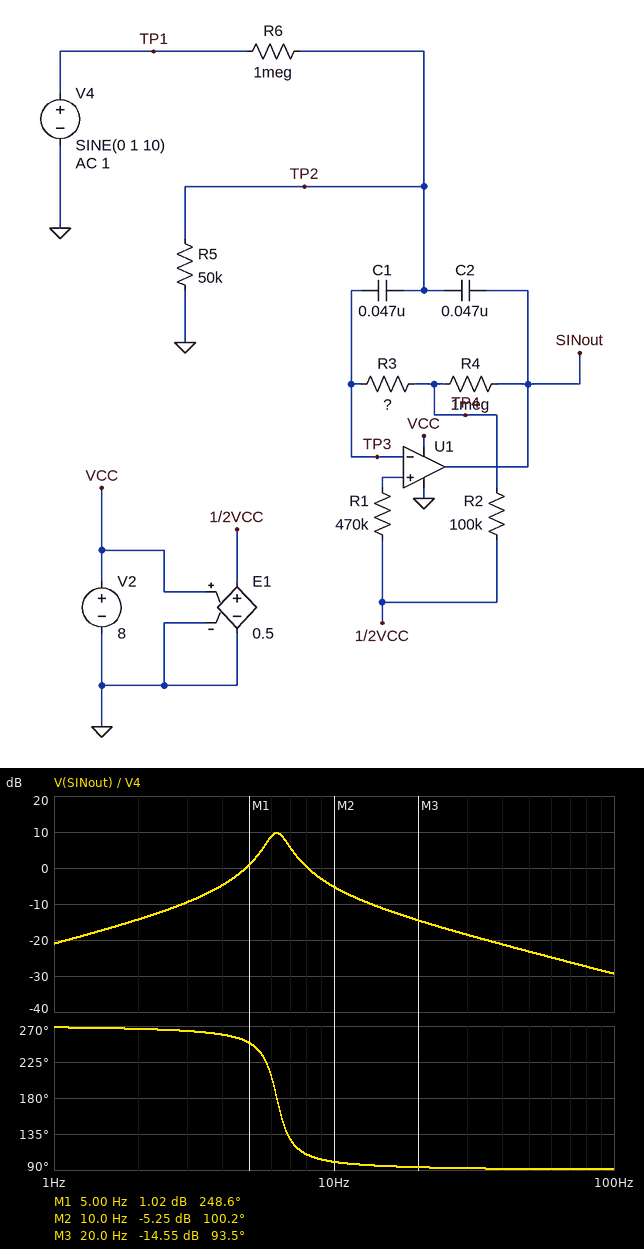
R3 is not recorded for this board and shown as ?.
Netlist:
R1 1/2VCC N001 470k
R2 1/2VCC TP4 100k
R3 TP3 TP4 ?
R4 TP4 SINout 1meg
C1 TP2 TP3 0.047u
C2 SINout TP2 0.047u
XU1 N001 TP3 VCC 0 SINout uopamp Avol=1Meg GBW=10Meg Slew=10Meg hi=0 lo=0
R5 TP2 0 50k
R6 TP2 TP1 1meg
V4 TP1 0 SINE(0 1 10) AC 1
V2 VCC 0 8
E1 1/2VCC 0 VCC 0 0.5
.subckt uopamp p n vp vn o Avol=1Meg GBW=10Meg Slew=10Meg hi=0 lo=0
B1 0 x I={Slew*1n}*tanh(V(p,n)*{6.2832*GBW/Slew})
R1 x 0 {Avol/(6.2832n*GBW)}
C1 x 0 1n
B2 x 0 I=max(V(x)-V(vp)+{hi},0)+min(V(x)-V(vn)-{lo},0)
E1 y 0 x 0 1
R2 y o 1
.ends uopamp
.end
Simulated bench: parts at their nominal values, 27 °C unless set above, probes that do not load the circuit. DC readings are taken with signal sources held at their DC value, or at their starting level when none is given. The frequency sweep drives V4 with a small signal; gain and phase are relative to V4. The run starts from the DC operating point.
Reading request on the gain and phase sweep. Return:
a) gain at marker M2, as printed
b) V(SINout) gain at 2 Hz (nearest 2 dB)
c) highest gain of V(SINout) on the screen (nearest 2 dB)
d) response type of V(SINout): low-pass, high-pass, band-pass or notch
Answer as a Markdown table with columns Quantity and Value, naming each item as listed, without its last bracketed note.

| Quantity | Value |
|---|---|
| gain at marker M2, as printed | -5.25 dB |
| V(SINout) gain at 2 Hz | -14 dB |
| highest gain of V(SINout) on the screen | 10 dB |
| response type of V(SINout): low-pass, high-pass, band-pass or notch | band-pass |
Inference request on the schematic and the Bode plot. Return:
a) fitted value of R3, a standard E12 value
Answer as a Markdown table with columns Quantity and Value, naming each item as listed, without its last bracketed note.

| Quantity | Value |
|---|---|
| fitted value of R3, a standard E12 value | 470 kΩ |
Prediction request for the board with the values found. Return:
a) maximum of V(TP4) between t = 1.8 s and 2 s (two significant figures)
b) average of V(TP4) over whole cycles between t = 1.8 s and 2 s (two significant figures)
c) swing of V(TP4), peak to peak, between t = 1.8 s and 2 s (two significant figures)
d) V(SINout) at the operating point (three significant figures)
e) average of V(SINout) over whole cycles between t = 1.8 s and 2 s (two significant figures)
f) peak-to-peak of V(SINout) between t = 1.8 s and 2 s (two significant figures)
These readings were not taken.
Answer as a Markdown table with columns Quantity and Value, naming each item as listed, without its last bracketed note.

| Quantity | Value |
|---|---|
| maximum of V(TP4) between t = 1.8 s and 2 s | 4.0 V |
| average of V(TP4) over whole cycles between t = 1.8 s and 2 s | 4.0 V |
| swing of V(TP4), peak to peak, between t = 1.8 s and 2 s | 83 mV |
| V(SINout) at the operating point | 4.00 V |
| average of V(SINout) over whole cycles between t = 1.8 s and 2 s | 4.0 V |
| peak-to-peak of V(SINout) between t = 1.8 s and 2 s | 1.1 V |
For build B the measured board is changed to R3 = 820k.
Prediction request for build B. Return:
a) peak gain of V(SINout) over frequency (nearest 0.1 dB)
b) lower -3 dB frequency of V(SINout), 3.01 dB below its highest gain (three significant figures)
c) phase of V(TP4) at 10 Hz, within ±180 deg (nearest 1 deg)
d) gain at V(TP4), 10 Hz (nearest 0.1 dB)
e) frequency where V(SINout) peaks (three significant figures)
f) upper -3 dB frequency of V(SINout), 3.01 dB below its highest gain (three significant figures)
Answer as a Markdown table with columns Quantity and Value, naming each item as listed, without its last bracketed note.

| Quantity | Value |
|---|---|
| peak gain of V(SINout) over frequency | 14.0 dB |
| lower -3 dB frequency of V(SINout), 3.01 dB below its highest gain | 4.58 Hz |
| phase of V(TP4) at 10 Hz, within ±180 deg | 95 deg |
| gain at V(TP4), 10 Hz | -28.8 dB |
| frequency where V(SINout) peaks | 4.90 Hz |
| upper -3 dB frequency of V(SINout), 3.01 dB below its highest gain | 5.25 Hz |
